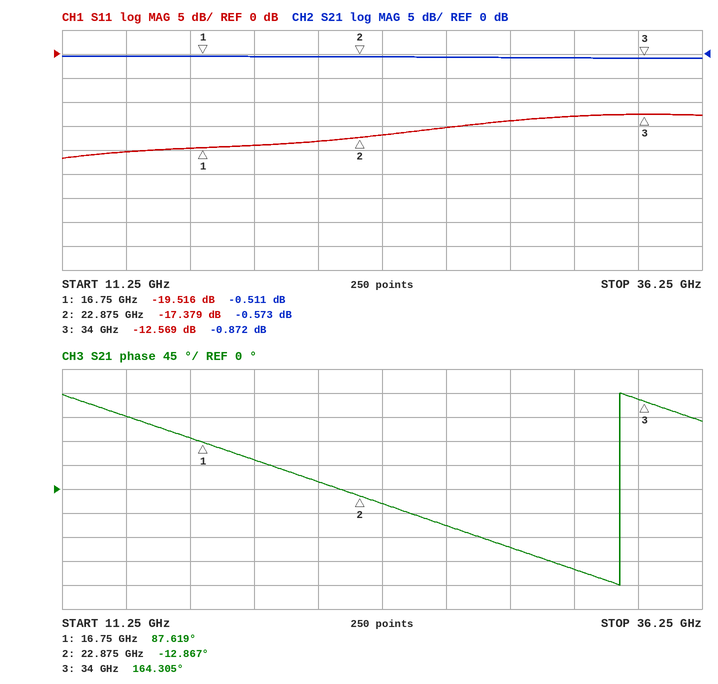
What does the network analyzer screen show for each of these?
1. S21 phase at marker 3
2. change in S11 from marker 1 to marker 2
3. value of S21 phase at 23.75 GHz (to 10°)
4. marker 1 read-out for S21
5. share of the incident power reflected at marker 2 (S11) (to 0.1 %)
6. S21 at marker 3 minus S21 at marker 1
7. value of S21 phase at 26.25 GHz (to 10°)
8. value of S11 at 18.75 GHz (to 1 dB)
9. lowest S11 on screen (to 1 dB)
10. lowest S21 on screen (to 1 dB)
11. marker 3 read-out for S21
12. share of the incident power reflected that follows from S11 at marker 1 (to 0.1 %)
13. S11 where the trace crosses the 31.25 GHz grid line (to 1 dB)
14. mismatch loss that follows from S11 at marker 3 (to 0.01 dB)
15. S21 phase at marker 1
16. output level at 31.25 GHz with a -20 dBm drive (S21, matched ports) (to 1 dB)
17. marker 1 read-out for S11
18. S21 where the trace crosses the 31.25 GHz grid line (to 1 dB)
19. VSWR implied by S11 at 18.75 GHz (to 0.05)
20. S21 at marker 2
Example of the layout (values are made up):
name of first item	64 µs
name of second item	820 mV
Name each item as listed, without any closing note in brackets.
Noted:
S21 phase at marker 3	164.305°
change in S11 from marker 1 to marker 2	2.137 dB
value of S21 phase at 23.75 GHz	-30°
marker 1 read-out for S21	-0.511 dB
share of the incident power reflected at marker 2 (S11)	1.8 %
S21 at marker 3 minus S21 at marker 1	-0.361 dB
value of S21 phase at 26.25 GHz	-70°
value of S11 at 18.75 GHz	-19 dB
lowest S11 on screen	-22 dB
lowest S21 on screen	-1 dB
marker 3 read-out for S21	-0.872 dB
share of the incident power reflected that follows from S11 at marker 1	1.1 %
S11 where the trace crosses the 31.25 GHz grid line	-13 dB
mismatch loss that follows from S11 at marker 3	0.25 dB
S21 phase at marker 1	87.619°
output level at 31.25 GHz with a -20 dBm drive (S21, matched ports)	-21 dBm
marker 1 read-out for S11	-19.516 dB
S21 where the trace crosses the 31.25 GHz grid line	-1 dB
VSWR implied by S11 at 18.75 GHz	1.25
S21 at marker 2	-0.573 dB
